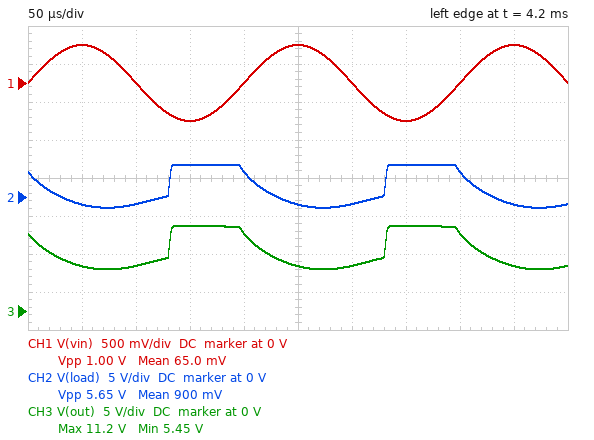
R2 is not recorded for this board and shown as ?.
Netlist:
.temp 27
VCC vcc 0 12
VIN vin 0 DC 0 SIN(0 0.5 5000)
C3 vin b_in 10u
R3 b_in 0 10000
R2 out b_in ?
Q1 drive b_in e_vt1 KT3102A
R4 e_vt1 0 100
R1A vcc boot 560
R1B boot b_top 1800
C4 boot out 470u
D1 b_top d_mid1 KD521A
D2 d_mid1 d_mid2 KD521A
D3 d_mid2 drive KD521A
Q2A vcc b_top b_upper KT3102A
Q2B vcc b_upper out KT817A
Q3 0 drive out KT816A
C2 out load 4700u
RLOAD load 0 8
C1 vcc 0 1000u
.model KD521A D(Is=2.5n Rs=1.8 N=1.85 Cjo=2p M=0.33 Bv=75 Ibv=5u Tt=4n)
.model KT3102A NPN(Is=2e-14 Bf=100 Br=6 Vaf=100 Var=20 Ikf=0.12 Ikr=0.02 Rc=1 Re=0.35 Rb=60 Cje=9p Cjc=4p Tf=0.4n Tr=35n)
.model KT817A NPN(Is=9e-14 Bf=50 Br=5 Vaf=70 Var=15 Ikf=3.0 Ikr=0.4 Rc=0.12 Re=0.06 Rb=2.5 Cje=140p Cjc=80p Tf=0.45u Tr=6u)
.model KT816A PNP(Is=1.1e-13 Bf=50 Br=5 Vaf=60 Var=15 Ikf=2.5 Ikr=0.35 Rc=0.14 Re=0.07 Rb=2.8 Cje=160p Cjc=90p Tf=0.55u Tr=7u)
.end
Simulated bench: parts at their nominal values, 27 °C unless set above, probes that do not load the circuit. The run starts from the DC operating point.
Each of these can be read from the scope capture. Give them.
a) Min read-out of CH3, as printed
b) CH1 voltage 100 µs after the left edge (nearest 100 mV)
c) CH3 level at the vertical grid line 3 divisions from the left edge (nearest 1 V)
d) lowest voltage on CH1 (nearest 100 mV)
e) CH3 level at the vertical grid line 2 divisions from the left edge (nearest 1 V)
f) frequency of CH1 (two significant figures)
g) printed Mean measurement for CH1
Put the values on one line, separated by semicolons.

5.45 V; 0 V; 11 V; -500 mV; 6 V; 5.0 kHz; 65.0 mV
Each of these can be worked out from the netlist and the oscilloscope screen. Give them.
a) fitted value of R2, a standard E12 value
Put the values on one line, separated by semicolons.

56 kΩ
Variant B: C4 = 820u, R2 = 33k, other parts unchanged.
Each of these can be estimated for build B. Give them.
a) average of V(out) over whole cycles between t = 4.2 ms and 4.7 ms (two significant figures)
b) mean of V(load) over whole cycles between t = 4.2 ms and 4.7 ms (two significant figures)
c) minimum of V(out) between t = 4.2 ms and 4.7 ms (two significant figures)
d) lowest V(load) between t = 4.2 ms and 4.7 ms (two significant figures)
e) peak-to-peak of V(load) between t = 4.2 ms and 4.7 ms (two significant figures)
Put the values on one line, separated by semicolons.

7.0 V; 1.7 V; 3.8 V; -1.5 V; 7.3 V
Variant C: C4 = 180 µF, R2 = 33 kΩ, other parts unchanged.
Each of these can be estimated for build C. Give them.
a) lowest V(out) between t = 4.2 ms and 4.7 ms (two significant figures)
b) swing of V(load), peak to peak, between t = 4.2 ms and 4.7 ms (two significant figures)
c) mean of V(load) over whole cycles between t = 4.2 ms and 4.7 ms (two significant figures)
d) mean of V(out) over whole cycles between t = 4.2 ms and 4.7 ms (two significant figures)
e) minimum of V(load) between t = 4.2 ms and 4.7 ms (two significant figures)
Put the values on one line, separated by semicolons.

3.8 V; 7.3 V; 1.7 V; 7.0 V; -1.5 V
